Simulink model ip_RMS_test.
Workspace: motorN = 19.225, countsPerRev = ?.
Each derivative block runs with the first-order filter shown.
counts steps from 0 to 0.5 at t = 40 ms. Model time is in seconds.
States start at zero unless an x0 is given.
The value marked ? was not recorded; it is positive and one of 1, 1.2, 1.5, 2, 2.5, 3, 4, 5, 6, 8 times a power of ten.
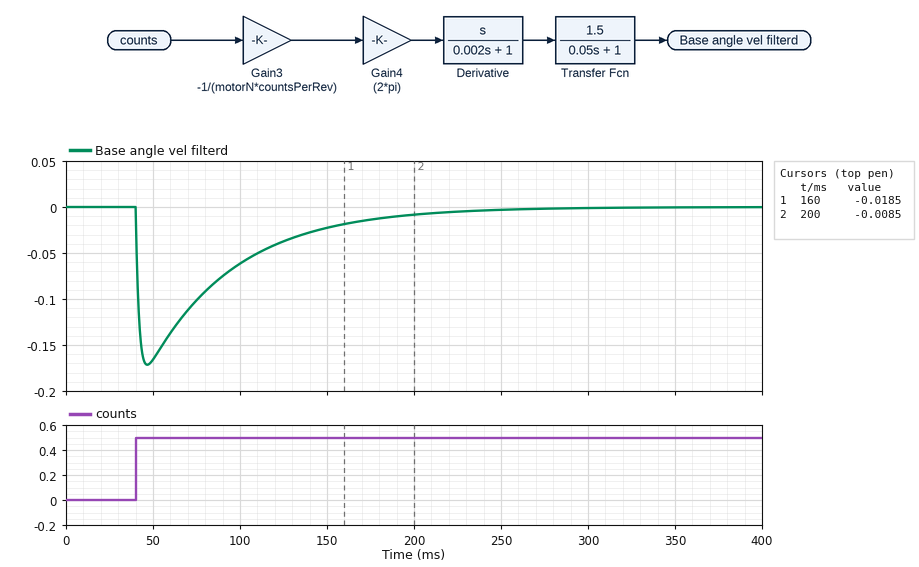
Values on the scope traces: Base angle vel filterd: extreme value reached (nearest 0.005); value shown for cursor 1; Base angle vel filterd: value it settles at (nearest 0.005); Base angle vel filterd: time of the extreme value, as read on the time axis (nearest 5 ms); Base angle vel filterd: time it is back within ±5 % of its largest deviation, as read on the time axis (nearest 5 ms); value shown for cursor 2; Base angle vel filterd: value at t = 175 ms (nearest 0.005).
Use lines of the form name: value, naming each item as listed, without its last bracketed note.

Base angle vel filterd: extreme value reached: -0.170
value shown for cursor 1: -0.0185
Base angle vel filterd: value it settles at: 0.000
Base angle vel filterd: time of the extreme value, as read on the time axis: 45 ms
Base angle vel filterd: time it is back within ±5 % of its largest deviation, as read on the time axis: 200 ms
value shown for cursor 2: -0.0085
Base angle vel filterd: value at t = 175 ms: -0.015
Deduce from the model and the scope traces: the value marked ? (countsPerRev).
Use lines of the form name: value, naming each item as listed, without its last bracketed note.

the value marked ?: 25
